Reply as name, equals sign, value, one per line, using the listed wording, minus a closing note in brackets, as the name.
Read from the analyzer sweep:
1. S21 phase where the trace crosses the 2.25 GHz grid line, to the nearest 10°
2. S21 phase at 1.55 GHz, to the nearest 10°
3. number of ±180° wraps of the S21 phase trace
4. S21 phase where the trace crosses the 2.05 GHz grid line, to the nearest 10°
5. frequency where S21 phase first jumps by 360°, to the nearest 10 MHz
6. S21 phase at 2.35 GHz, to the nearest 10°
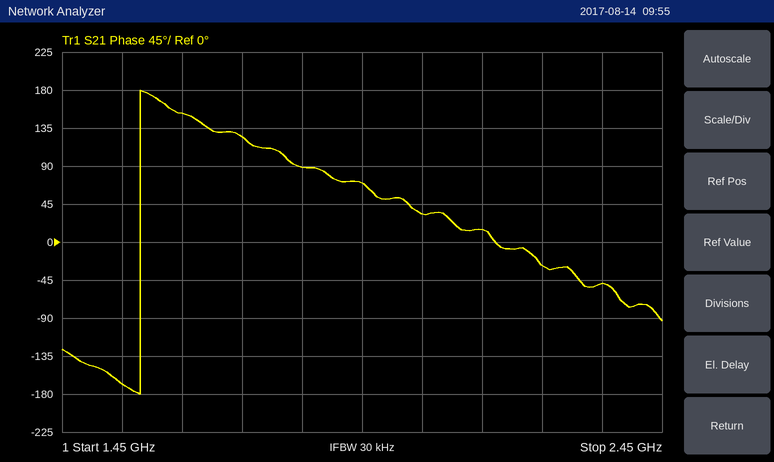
S21 phase where the trace crosses the 2.25 GHz grid line, to the nearest 10° = -30°
S21 phase at 1.55 GHz, to the nearest 10° = -170°
number of ±180° wraps of the S21 phase trace = 1
S21 phase where the trace crosses the 2.05 GHz grid line, to the nearest 10° = 30°
frequency where S21 phase first jumps by 360°, to the nearest 10 MHz = 1.58 GHz
S21 phase at 2.35 GHz, to the nearest 10° = -50°
